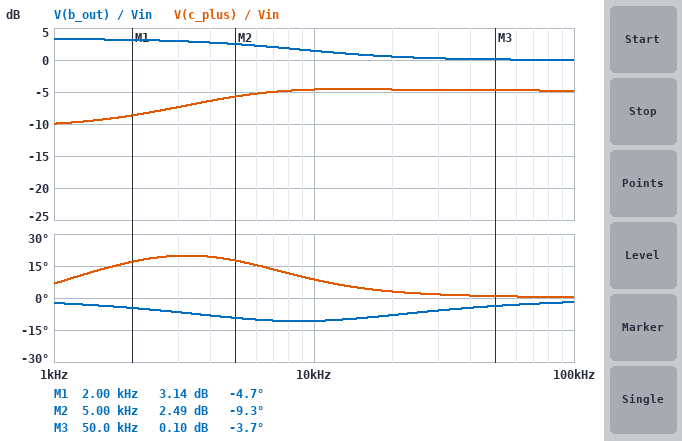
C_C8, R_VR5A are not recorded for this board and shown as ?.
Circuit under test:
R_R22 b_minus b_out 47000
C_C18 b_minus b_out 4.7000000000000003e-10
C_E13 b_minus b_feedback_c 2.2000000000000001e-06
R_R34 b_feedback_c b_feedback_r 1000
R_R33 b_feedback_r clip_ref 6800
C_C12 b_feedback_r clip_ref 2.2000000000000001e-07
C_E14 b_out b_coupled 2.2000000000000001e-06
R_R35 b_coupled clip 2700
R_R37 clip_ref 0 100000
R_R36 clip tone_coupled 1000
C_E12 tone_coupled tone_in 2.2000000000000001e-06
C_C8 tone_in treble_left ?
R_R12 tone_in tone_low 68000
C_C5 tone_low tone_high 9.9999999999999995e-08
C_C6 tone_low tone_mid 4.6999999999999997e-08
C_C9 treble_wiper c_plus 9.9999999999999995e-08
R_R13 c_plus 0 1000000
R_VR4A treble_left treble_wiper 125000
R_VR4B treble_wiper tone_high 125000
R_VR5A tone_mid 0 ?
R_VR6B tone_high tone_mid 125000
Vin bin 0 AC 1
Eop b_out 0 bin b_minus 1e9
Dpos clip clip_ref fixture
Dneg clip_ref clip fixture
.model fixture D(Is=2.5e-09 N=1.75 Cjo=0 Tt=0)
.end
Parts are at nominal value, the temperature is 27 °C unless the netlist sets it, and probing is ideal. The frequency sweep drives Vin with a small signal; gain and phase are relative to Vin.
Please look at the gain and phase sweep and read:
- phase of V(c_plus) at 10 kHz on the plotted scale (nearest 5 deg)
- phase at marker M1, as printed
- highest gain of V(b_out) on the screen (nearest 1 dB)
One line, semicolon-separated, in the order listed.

10 deg; -4.7 deg; 3 dB
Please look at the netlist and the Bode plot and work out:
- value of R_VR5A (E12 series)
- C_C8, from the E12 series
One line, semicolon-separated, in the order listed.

22 kΩ; 100 pF
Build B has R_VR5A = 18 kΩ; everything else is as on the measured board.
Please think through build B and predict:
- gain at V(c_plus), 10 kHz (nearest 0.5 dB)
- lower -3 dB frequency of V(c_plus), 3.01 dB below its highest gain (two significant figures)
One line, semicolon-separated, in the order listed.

-5.0 dB; 7.1 Hz
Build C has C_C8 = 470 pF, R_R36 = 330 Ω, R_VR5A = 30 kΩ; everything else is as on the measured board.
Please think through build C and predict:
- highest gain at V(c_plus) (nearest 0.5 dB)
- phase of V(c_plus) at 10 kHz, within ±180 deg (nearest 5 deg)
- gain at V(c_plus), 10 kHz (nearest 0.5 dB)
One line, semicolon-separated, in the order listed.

-2.0 dB; -5 deg; -3.0 dB
